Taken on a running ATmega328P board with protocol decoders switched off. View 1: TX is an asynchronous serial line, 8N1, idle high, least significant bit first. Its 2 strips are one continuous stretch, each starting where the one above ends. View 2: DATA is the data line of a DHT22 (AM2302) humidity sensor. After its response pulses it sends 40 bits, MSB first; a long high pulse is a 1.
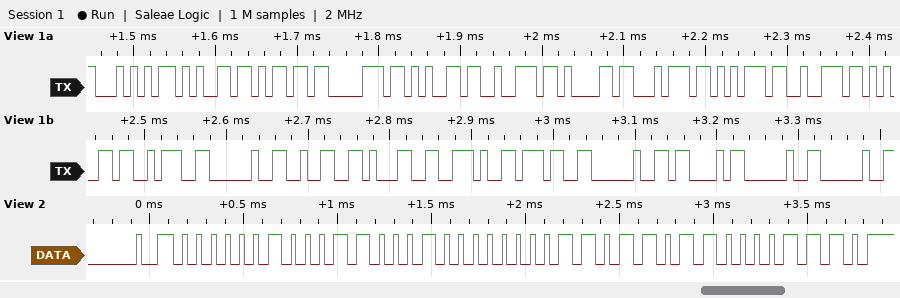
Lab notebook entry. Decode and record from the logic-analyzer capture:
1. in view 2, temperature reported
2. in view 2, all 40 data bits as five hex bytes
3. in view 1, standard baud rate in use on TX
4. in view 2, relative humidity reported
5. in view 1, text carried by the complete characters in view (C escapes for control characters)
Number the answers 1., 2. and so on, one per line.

1. 21.9 °C
2. 02 31 00 DB 0E
3. 115200 baud
4. 56.1 %
5. "Temperature: 21.7 C  "
